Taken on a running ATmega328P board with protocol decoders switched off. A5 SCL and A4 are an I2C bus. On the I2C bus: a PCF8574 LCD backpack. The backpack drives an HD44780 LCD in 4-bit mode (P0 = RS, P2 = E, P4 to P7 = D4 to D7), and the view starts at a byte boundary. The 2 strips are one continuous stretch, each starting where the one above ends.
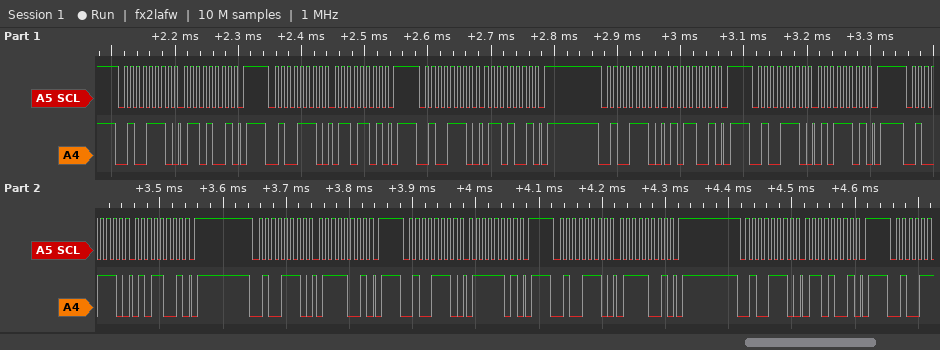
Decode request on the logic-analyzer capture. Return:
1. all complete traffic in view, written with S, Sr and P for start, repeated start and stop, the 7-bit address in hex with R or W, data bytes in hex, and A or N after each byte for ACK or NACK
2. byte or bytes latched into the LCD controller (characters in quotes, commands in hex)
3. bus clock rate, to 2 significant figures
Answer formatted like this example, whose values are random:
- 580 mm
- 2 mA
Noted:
- S 27W A 69 A P S 27W A 6D A P S 27W A 69 A P S 27W A 59 A P S 27W A 5D A P S 27W A 59 A P S 27W A 79 A P S 27W A 7D A P S 27W A 79 A P S 27W A 69 A P
- 'e'
- 100 kHz
